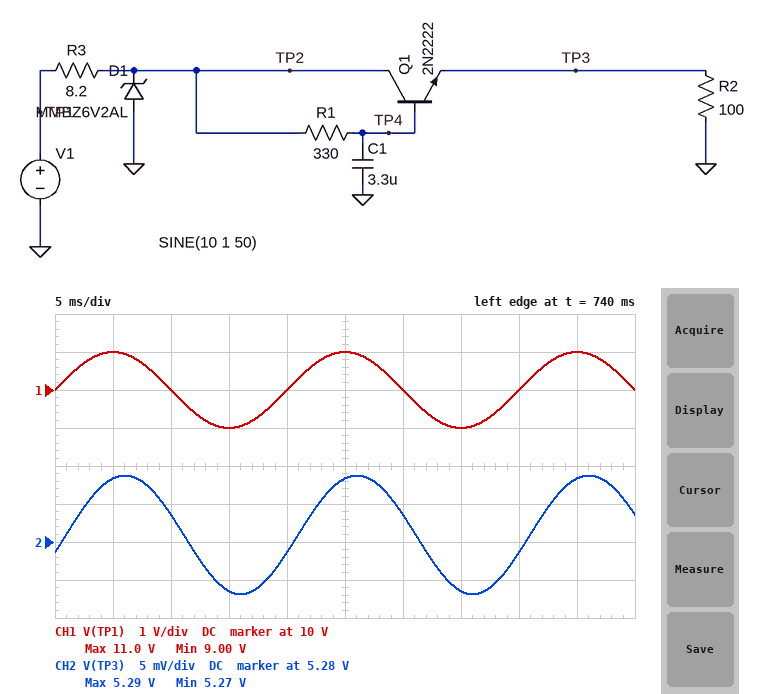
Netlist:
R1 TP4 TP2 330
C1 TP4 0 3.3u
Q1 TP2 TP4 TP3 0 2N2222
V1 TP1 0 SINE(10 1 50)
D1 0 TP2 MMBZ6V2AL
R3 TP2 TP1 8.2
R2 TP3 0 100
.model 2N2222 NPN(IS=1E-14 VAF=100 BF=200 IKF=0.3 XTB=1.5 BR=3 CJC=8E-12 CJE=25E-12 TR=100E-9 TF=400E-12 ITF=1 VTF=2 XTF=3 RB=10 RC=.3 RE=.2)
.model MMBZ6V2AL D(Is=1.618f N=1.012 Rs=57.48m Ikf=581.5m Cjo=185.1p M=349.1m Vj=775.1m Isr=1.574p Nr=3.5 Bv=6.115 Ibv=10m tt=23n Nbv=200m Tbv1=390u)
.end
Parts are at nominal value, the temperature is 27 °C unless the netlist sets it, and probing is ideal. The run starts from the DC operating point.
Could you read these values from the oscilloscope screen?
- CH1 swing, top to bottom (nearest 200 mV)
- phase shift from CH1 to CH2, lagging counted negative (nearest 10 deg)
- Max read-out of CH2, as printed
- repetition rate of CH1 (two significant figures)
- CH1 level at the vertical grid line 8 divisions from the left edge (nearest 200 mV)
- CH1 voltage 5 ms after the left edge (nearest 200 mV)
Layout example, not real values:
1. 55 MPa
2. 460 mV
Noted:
1. 2.0 V
2. -20 deg
3. 5.29 V
4. 50 Hz
5. 10.0 V
6. 11.0 V
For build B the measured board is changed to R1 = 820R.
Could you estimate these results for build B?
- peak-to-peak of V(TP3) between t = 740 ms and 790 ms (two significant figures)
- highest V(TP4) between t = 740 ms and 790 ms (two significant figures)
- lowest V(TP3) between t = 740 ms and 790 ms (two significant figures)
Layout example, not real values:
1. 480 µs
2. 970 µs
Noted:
1. 12 mV
2. 5.9 V
3. 5.1 V
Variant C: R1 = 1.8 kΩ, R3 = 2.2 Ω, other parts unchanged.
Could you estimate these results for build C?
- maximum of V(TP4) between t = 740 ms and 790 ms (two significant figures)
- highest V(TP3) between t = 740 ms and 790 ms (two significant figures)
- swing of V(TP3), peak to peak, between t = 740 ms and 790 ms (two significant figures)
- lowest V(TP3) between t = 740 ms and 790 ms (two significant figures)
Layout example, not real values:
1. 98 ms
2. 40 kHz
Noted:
1. 5.7 V
2. 5.0 V
3. 25 mV
4. 4.9 V
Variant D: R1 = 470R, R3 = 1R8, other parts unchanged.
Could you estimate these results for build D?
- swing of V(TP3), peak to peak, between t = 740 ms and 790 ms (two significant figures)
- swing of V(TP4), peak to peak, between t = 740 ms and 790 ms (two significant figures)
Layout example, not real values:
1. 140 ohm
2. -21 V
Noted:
1. 56 mV
2. 57 mV
